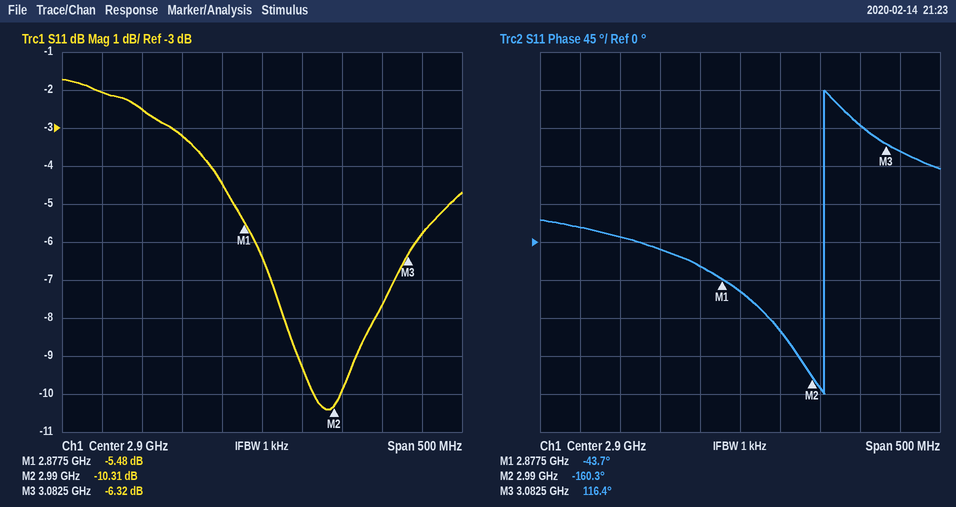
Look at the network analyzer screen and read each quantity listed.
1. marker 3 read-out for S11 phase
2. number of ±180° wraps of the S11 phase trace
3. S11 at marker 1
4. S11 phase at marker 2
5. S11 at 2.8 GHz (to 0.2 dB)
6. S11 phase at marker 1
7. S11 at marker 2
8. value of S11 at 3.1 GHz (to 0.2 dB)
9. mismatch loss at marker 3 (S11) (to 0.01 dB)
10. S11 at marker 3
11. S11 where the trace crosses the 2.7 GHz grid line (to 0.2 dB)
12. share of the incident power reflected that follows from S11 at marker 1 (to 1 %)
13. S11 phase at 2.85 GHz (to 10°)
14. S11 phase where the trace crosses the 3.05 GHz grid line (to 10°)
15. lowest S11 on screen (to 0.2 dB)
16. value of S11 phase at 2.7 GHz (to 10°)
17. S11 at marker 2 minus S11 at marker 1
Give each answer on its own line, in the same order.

116.4°
1
-5.48 dB
-160.3°
-3.2 dB
-43.7°
-10.31 dB
-5.8 dB
1.15 dB
-6.32 dB
-2.0 dB
28 %
-30°
140°
-10.4 dB
20°
-4.83 dB
